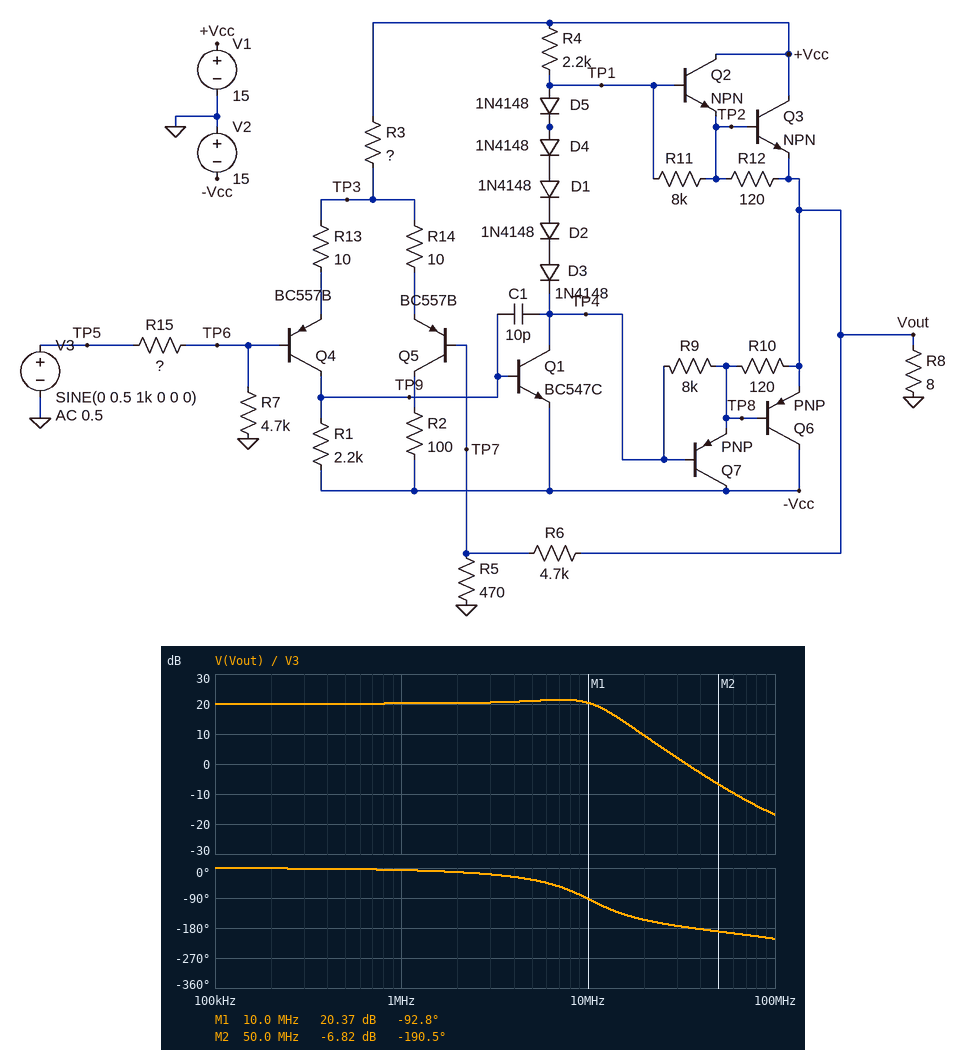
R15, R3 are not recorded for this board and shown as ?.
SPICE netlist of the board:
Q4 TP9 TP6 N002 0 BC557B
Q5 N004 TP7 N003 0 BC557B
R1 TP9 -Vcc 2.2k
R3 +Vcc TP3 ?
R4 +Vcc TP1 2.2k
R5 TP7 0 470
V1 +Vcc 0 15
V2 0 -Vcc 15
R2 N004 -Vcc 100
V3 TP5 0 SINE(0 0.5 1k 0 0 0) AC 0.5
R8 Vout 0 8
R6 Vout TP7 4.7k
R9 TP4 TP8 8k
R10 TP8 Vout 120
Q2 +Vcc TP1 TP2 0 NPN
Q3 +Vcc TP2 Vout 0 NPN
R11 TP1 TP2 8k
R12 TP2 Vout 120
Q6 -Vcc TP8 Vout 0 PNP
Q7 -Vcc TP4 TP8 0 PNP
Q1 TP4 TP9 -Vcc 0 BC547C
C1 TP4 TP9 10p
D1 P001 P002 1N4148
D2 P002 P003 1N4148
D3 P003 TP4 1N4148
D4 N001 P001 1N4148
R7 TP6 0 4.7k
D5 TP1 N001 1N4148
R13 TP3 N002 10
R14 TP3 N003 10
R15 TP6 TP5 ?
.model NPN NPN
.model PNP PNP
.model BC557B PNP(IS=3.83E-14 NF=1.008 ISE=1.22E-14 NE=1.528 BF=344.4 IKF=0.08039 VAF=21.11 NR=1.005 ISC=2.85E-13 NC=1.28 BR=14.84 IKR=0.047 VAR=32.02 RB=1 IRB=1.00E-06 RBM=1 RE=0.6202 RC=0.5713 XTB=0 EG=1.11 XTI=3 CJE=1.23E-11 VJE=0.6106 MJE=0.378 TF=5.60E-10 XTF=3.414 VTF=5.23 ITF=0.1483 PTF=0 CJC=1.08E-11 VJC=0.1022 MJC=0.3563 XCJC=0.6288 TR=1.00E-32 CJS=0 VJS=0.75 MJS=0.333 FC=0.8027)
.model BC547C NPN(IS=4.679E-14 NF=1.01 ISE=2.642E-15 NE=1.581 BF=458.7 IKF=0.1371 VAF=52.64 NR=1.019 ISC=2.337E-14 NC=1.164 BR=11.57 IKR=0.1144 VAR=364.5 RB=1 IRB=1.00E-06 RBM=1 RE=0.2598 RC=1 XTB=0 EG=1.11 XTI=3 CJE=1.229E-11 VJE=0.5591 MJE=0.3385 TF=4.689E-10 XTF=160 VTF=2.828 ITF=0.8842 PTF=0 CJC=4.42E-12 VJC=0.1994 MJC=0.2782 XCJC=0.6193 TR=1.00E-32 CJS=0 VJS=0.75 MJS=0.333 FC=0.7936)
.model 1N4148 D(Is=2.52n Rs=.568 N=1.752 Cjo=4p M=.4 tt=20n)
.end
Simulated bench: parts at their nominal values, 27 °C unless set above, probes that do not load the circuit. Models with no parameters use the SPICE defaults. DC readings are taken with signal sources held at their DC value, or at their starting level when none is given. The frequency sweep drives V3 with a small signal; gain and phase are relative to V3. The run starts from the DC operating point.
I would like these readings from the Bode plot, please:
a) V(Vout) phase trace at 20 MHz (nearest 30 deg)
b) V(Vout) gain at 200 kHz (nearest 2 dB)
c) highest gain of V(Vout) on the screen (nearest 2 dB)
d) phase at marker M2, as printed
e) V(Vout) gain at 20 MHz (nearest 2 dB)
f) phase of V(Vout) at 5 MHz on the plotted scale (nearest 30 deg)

-150 deg
20 dB
22 dB
-190.5 deg
10 dB
-30 deg
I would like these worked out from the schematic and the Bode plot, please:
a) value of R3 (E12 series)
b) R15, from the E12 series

8.2 kΩ
390 Ω
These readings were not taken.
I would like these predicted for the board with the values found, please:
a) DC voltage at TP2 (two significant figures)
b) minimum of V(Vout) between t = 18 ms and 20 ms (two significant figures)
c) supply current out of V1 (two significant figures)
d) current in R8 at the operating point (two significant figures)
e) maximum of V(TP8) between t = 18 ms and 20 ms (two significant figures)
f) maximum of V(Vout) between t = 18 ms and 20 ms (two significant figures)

240 mV
-5.7 V
19 mA
72 mA
3.9 V
4.5 V
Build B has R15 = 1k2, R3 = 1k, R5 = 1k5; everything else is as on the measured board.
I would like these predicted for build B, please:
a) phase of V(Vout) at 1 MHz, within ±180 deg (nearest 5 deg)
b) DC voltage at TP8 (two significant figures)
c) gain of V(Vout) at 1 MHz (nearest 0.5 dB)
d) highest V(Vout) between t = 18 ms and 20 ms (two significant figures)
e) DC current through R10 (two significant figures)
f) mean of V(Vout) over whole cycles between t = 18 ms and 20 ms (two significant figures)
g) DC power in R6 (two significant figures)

0 deg
-2.1 V
10.5 dB
510 mV
7.5 mA
-1.2 V
180 µW
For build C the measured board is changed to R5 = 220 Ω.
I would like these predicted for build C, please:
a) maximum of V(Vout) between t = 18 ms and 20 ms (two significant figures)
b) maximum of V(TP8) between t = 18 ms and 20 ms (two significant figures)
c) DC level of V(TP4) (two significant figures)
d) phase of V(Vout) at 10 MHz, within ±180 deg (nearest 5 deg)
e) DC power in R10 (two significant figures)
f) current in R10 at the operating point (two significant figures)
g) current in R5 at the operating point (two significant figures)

9.1 V
8.7 V
-2.9 V
-110 deg
6.8 mW
7.5 mA
230 µA
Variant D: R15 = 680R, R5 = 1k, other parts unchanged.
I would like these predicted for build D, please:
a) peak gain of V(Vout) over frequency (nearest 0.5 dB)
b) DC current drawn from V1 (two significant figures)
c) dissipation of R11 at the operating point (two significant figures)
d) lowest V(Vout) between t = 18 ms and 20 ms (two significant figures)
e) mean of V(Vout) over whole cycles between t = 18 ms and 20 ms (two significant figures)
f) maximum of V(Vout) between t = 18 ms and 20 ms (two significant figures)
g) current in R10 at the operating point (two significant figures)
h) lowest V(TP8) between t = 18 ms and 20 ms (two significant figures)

20.5 dB
21 mA
85 µW
-2.8 V
-300 mV
2.2 V
7.3 mA
-3.7 V
